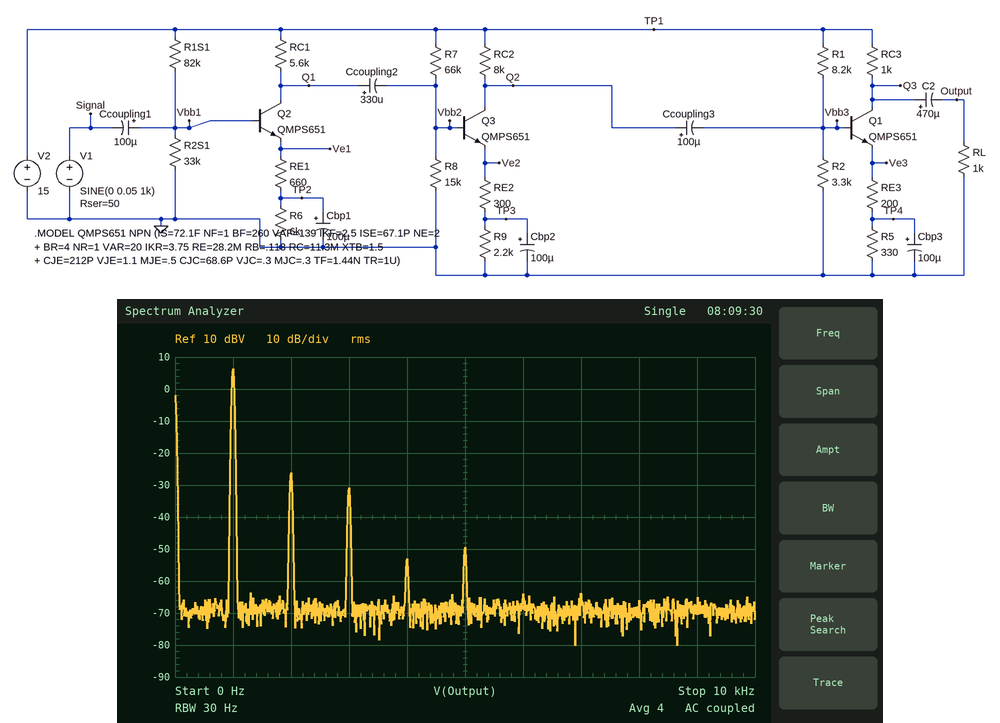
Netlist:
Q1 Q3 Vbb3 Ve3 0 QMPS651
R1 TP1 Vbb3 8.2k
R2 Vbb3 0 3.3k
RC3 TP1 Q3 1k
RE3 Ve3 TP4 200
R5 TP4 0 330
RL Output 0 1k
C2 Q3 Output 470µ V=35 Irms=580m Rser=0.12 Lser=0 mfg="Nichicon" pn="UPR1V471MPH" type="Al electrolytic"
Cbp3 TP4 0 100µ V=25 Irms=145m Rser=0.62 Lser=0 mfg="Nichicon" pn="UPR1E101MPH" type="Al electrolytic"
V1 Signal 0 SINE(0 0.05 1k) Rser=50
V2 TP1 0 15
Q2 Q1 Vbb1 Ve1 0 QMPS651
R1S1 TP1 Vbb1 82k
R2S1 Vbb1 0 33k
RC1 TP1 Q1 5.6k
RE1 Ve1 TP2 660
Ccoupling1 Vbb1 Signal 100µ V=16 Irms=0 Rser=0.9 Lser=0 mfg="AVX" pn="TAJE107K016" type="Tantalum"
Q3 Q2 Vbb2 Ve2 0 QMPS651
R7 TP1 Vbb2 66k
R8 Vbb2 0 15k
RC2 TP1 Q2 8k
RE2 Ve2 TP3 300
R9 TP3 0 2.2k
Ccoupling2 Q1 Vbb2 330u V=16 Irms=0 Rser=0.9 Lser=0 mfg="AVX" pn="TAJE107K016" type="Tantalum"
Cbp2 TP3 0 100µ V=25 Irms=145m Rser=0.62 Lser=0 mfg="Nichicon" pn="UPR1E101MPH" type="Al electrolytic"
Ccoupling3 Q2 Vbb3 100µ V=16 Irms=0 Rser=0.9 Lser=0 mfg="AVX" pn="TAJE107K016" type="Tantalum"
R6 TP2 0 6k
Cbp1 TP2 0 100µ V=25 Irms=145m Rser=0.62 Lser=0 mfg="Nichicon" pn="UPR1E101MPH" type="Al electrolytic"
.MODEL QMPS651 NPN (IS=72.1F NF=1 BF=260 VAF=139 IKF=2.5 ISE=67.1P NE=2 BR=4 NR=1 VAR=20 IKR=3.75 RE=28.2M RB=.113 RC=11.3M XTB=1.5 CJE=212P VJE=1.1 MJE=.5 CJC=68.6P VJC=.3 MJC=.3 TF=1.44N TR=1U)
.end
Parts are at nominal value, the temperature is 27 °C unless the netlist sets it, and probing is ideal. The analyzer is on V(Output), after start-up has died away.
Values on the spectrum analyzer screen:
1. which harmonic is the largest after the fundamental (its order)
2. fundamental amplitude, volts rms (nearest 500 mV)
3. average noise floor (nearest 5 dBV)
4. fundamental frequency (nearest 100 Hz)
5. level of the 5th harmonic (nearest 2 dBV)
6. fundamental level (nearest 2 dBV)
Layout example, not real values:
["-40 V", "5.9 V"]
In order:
["2", "2.0 V", "-70 dBV", "1.0 kHz", "-50 dBV", "6 dBV"]
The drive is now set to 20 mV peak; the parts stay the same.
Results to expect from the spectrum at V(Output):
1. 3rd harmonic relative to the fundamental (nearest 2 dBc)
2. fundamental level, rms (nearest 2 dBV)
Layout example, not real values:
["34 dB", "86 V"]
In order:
["-58 dBc", "-2 dBV"]
